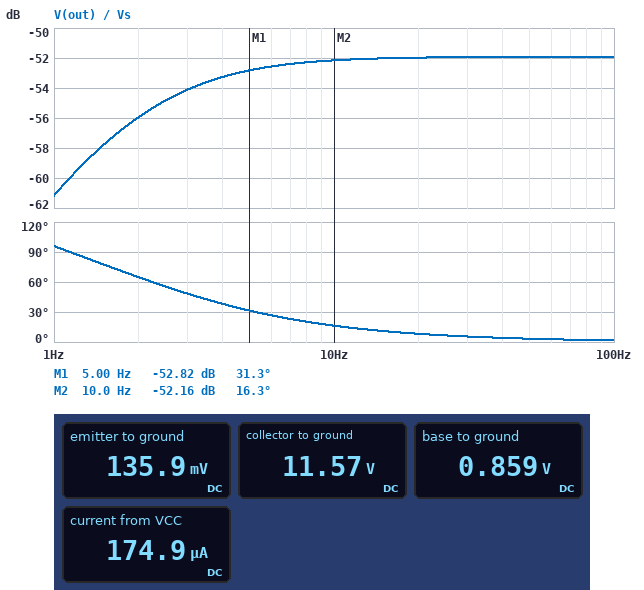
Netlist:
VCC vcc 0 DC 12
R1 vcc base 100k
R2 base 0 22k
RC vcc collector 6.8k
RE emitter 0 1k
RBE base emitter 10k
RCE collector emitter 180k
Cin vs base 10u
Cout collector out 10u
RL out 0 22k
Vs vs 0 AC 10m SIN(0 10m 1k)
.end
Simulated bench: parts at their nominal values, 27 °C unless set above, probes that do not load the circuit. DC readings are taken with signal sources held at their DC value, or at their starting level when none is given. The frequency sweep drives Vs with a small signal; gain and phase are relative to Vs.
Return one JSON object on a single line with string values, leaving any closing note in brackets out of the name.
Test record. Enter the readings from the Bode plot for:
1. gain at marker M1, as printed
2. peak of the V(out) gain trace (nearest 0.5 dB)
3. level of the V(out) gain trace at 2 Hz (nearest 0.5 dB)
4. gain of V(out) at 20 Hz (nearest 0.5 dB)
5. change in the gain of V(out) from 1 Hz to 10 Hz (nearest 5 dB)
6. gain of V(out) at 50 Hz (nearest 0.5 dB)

{"gain at marker M1, as printed": "-52.82 dB", "peak of the V(out) gain trace": "-52.0 dB", "level of the V(out) gain trace at 2 Hz": "-56.0 dB", "gain of V(out) at 20 Hz": "-52.0 dB", "change in the gain of V(out) from 1 Hz to 10 Hz": "10 dB", "gain of V(out) at 50 Hz": "-52.0 dB"}
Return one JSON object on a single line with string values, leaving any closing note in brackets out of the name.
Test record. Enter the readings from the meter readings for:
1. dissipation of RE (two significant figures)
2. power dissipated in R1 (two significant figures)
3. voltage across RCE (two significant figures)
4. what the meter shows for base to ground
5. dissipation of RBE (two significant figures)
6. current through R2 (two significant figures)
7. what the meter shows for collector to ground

{"dissipation of RE": "18 µW", "power dissipated in R1": "1.2 mW", "voltage across RCE": "11 V", "what the meter shows for base to ground": "0.859 V", "dissipation of RBE": "52 µW", "current through R2": "39 µA", "what the meter shows for collector to ground": "11.57 V"}
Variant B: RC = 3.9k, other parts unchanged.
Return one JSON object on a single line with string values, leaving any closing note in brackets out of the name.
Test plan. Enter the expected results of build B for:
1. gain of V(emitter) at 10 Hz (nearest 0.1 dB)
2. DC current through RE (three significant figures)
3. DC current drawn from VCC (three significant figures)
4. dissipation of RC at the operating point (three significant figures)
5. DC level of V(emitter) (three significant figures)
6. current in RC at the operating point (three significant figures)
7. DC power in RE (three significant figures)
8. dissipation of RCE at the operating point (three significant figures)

{"gain of V(emitter) at 10 Hz": "-21.1 dB", "DC current through RE": "137 µA", "DC current drawn from VCC": "176 µA", "dissipation of RC at the operating point": "16.2 µW", "DC level of V(emitter)": "137 mV", "current in RC at the operating point": "64.5 µA", "DC power in RE": "18.7 µW", "dissipation of RCE at the operating point": "749 µW"}
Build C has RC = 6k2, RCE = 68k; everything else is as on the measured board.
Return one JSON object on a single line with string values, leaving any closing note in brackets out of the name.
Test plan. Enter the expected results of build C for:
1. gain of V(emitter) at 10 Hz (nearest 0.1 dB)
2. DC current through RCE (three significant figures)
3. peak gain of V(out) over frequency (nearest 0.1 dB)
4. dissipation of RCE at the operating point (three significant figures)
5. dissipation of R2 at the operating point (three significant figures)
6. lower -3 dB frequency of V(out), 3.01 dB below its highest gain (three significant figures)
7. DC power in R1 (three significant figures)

{"gain of V(emitter) at 10 Hz": "-21.2 dB", "DC current through RCE": "159 µA", "peak gain of V(out) over frequency": "-44.5 dB", "dissipation of RCE at the operating point": "1.71 mW", "dissipation of R2 at the operating point": "38.3 µW", "lower -3 dB frequency of V(out), 3.01 dB below its highest gain": "2.46 Hz", "DC power in R1": "1.23 mW"}
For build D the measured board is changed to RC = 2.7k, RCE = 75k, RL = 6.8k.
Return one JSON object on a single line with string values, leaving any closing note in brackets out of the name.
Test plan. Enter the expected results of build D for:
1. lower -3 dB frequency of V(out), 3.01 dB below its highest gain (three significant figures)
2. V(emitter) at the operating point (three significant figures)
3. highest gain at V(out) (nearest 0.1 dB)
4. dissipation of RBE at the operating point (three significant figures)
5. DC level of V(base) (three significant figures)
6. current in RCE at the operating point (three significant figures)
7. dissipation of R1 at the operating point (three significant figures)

{"lower -3 dB frequency of V(out), 3.01 dB below its highest gain": "3.14 Hz", "V(emitter) at the operating point": "221 mV", "highest gain at V(out)": "-52.9 dB", "dissipation of RBE at the operating point": "48.0 µW", "DC level of V(base)": "914 mV", "current in RCE at the operating point": "152 µA", "dissipation of R1 at the operating point": "1.23 mW"}
